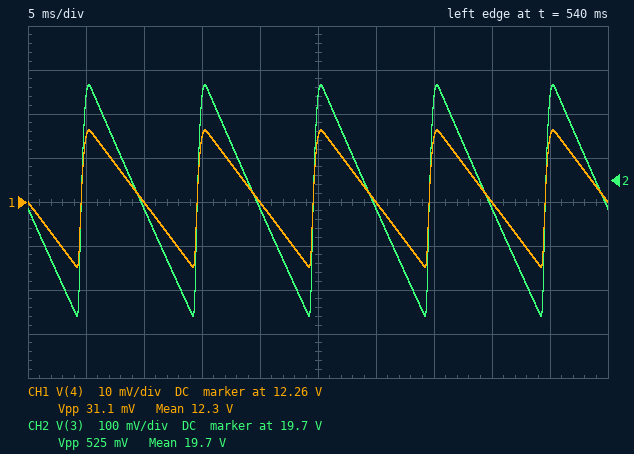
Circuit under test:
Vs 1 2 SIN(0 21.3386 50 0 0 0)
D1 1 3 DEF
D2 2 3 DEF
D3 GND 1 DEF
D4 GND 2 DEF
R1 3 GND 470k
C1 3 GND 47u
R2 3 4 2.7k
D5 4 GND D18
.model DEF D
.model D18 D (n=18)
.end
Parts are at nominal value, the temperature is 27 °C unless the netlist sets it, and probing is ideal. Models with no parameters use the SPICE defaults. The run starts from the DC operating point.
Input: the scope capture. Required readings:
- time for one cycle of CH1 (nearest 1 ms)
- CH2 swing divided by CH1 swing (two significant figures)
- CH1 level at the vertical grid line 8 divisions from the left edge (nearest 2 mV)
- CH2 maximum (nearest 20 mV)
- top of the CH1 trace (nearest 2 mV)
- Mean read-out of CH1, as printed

10 ms
17
12.260 V
19.92 V
12.276 V
12.3 V
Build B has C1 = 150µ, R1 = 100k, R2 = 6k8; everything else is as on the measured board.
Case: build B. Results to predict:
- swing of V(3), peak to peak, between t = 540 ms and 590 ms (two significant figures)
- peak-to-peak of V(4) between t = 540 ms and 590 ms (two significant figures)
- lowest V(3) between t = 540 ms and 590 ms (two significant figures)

83 mV
4.6 mV
20 V
